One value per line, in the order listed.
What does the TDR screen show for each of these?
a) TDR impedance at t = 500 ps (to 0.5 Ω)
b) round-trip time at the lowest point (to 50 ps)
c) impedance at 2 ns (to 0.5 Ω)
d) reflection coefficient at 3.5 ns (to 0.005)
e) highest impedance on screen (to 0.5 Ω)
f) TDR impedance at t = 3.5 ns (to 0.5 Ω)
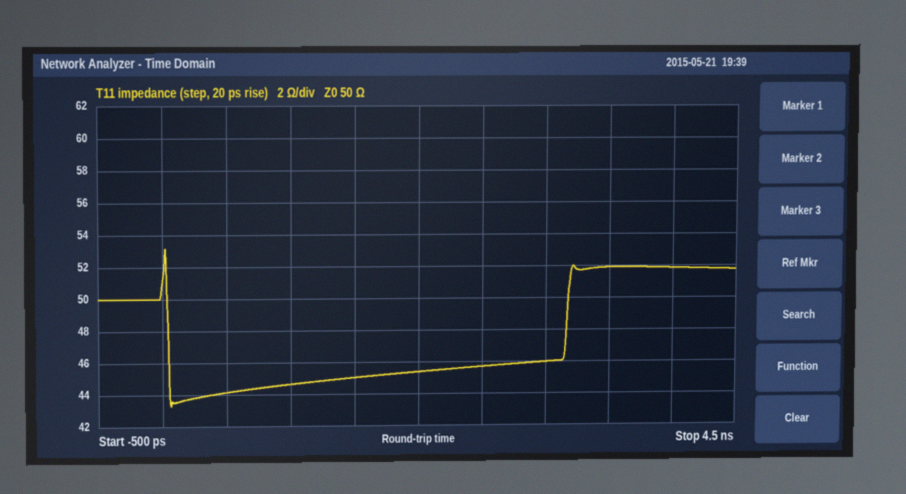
44.0 Ω
50 ps
45.5 Ω
+0.020
53.0 Ω
52.0 Ω
